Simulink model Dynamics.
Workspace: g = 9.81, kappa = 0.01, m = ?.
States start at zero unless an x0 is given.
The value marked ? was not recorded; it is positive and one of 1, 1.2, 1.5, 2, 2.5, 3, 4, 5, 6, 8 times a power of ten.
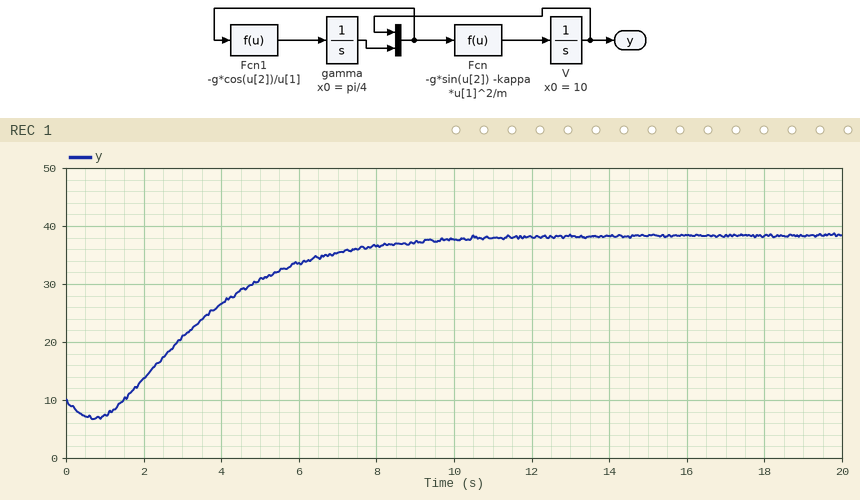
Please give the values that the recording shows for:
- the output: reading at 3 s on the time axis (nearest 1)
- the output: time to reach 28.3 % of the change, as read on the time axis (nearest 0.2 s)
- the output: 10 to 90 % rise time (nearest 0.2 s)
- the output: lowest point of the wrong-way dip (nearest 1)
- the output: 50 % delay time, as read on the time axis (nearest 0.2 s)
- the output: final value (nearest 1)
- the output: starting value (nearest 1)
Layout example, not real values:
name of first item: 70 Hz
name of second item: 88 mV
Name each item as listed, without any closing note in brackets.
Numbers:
the output: reading at 3 s on the time axis: 21
the output: time to reach 28.3 % of the change, as read on the time axis: 2.6 s
the output: 10 to 90 % rise time: 5.2 s
the output: lowest point of the wrong-way dip: 7
the output: 50 % delay time, as read on the time axis: 3.6 s
the output: final value: 38
the output: starting value: 10
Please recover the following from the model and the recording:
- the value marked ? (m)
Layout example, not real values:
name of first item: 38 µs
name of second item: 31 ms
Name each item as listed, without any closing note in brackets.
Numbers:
the value marked ?: 1.5
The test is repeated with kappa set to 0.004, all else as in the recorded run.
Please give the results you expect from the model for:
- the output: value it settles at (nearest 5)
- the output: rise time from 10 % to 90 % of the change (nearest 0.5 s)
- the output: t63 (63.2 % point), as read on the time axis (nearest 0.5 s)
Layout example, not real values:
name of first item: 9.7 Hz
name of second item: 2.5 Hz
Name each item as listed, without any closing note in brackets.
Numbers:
the output: value it settles at: 60
the output: rise time from 10 % to 90 % of the change: 8.5 s
the output: t63 (63.2 % point), as read on the time axis: 6.0 s
